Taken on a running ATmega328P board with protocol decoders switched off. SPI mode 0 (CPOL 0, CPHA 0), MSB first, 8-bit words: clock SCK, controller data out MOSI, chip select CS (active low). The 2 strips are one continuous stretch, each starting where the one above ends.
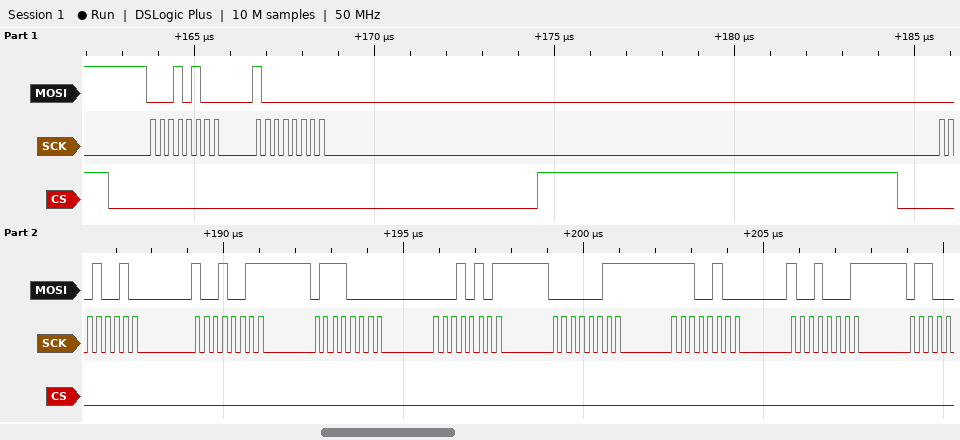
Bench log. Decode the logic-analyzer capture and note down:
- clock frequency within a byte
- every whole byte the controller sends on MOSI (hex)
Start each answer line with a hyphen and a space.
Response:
- 4 MHz
- 14 80 12 93 70 15 03 E4 91
